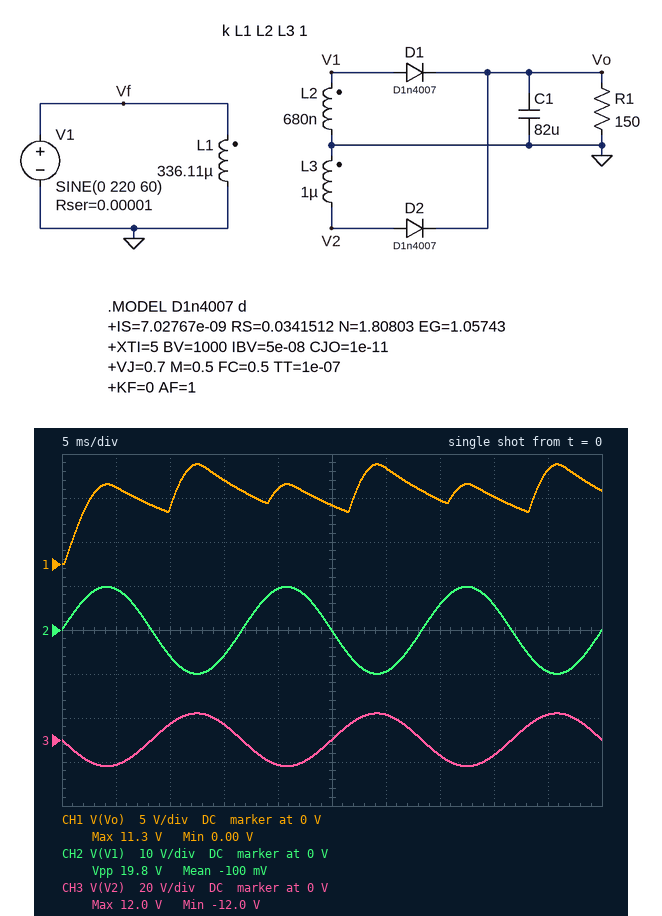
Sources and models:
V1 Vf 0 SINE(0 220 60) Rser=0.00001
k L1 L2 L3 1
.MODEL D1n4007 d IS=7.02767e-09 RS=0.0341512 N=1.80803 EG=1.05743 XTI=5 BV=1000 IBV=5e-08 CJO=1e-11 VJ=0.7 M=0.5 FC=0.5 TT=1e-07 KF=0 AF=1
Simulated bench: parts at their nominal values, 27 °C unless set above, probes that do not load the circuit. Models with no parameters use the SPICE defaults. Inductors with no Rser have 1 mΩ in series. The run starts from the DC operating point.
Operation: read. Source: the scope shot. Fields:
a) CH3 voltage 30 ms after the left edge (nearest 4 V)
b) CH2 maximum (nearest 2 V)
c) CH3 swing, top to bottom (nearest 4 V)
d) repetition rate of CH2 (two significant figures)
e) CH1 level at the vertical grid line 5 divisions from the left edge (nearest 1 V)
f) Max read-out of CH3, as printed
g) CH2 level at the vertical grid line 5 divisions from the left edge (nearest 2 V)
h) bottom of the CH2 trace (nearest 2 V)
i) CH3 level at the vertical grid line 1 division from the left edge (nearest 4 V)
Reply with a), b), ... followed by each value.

a) 12 V
b) 10 V
c) 24 V
d) 60 Hz
e) 7 V
f) 12.0 V
g) 0 V
h) -10 V
i) -12 V
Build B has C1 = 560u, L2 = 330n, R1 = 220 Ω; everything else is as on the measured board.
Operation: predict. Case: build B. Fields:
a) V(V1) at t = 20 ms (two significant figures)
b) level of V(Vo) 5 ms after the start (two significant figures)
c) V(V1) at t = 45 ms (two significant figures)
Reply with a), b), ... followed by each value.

a) 6.5 V
b) 6.1 V
c) -6.6 V
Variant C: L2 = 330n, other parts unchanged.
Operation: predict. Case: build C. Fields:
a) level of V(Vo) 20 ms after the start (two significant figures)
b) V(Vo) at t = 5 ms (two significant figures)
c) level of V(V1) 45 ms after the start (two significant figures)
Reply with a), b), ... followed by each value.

a) 6.3 V
b) 5.9 V
c) -6.6 V
